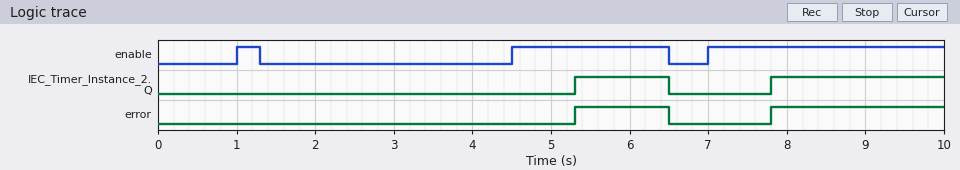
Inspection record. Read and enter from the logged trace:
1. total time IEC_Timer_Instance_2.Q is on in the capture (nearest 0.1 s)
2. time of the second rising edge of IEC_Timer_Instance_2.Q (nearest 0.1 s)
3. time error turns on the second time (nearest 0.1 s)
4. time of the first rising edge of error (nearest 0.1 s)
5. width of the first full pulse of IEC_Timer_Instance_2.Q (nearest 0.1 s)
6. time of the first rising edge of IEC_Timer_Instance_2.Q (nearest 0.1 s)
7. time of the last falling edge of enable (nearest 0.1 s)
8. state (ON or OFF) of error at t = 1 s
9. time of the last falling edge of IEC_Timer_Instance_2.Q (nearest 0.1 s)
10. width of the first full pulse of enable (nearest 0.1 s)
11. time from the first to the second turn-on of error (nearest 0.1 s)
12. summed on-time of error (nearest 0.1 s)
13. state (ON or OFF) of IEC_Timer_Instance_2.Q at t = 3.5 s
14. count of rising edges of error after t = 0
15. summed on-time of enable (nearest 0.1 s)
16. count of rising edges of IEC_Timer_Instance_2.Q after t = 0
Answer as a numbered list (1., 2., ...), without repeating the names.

1. 3.4 s
2. 7.8 s
3. 7.8 s
4. 5.3 s
5. 1.2 s
6. 5.3 s
7. 6.5 s
8. OFF
9. 6.5 s
10. 0.3 s
11. 2.5 s
12. 3.4 s
13. OFF
14. 2
15. 5.3 s
16. 2
